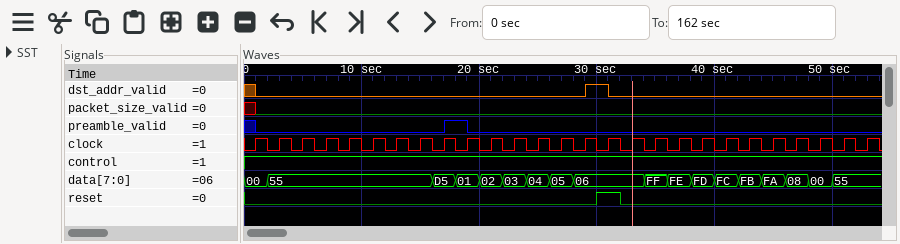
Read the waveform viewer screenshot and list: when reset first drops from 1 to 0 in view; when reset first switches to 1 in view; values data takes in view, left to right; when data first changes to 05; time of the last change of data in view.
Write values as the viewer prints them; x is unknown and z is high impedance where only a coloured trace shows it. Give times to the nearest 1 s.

32 s
30 s
00, 55, D5, 01, 02, 03, 04, 05, 06, FF, FE, FD, FC, FB, FA, 08, 00, 55
26 s
50 s
